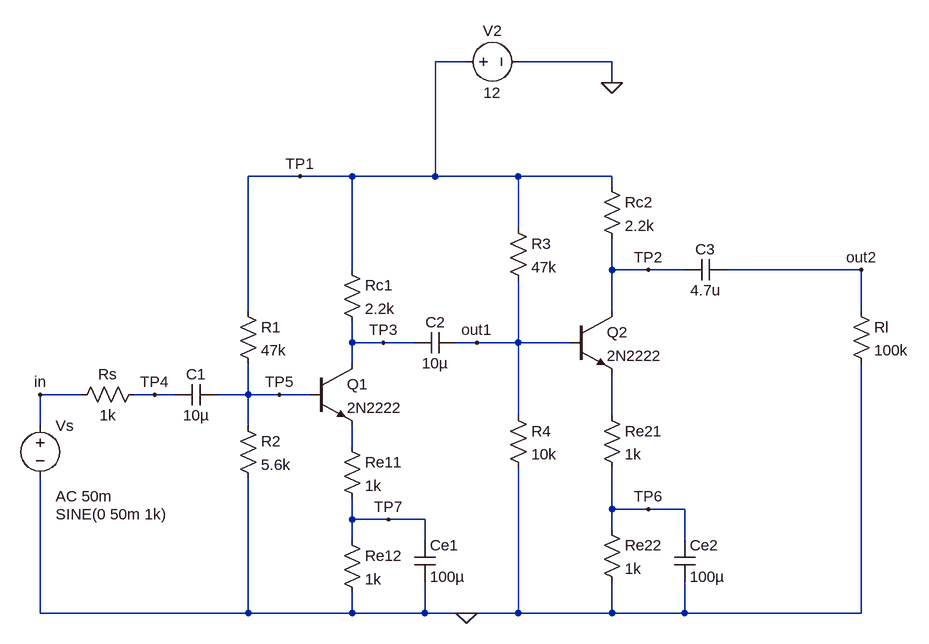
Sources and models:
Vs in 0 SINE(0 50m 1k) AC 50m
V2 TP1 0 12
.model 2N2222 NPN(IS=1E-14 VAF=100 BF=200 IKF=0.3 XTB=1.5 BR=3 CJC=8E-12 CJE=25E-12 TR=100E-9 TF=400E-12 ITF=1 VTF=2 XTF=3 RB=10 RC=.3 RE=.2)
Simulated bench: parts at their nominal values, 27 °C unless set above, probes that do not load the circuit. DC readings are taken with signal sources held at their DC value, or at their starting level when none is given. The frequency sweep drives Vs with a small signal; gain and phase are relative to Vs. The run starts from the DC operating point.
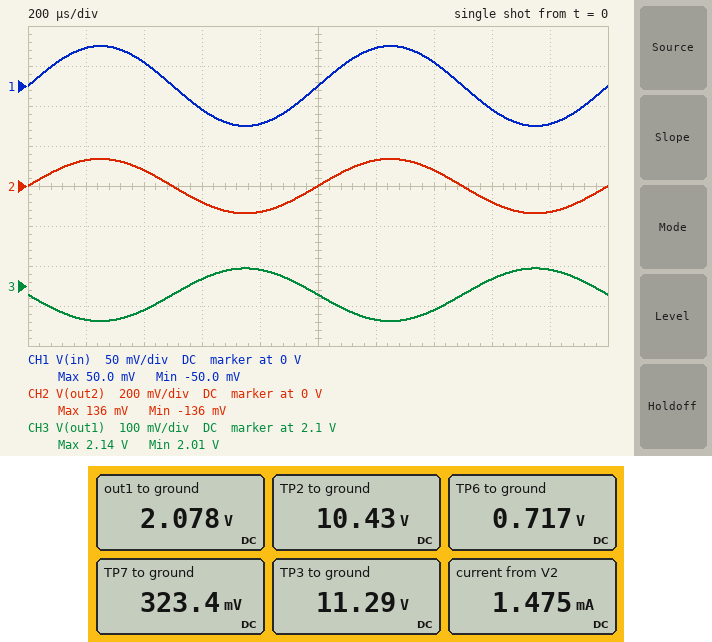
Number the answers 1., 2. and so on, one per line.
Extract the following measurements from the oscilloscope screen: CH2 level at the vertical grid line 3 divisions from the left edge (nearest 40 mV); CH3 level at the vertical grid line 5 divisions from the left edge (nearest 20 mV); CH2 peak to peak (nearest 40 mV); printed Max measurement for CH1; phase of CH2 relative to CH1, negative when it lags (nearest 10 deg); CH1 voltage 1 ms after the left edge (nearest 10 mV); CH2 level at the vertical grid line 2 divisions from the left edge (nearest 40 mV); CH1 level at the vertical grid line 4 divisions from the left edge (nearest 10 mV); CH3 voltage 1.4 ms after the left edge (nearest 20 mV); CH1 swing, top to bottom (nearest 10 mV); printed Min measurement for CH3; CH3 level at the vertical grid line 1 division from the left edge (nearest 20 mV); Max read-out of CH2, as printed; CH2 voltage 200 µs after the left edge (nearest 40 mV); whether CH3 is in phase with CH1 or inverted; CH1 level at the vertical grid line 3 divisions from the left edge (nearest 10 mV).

1. -80 mV
2. 2.08 V
3. 280 mV
4. 50.0 mV
5. 0 deg
6. 0 V
7. 80 mV
8. -50 mV
9. 2.04 V
10. 100 mV
11. 2.01 V
12. 2.02 V
13. 136 mV
14. 120 mV
15. inverted
16. -30 mV
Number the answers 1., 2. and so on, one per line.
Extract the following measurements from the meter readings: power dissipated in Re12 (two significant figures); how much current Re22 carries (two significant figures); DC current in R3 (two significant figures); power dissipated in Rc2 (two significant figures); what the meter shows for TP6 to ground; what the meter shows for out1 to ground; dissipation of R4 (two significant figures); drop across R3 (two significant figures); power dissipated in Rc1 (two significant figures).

1. 100 µW
2. 720 µA
3. 210 µA
4. 1.1 mW
5. 0.717 V
6. 2.078 V
7. 430 µW
8. 9.9 V
9. 230 µW
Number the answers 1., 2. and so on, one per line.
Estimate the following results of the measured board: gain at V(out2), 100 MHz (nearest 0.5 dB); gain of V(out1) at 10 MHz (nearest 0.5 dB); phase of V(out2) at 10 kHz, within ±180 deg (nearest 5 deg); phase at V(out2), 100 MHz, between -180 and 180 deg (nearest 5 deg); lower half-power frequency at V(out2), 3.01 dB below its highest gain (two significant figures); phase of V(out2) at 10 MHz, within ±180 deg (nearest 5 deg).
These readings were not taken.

1. -11.5 dB
2. -5.5 dB
3. 0 deg
4. 45 deg
5. 5.5 Hz
6. -130 deg
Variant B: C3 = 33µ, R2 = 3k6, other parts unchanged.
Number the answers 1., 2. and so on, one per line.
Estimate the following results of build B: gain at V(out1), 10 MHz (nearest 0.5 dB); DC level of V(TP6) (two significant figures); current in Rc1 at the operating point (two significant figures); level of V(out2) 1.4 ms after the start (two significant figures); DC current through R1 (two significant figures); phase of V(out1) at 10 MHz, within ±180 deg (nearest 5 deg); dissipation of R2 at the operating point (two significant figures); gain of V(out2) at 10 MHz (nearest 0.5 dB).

1. -7.5 dB
2. 720 mV
3. 130 µA
4. 65 mV
5. 240 µA
6. 80 deg
7. 200 µW
8. -2.0 dB
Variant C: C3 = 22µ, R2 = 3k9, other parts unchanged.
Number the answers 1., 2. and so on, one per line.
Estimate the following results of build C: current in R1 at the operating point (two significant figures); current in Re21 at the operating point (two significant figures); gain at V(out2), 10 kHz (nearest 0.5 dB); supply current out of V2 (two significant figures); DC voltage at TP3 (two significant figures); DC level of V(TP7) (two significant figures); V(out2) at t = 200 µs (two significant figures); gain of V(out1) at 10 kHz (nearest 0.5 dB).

1. 240 µA
2. 720 µA
3. 7.5 dB
4. 1.3 mA
5. 12 V
6. 160 mV
7. 110 mV
8. 1.0 dB
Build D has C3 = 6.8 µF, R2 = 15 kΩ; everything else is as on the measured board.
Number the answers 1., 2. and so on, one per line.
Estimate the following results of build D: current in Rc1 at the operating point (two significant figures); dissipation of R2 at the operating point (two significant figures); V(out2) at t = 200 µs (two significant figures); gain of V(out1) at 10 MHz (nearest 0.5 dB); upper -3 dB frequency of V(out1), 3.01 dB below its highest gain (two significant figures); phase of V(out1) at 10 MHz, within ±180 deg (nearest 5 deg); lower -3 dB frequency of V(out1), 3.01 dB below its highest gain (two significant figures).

1. 1.1 mA
2. 540 µW
3. 150 mV
4. -4.5 dB
5. 4.0 MHz
6. 100 deg
7. 3.6 Hz
